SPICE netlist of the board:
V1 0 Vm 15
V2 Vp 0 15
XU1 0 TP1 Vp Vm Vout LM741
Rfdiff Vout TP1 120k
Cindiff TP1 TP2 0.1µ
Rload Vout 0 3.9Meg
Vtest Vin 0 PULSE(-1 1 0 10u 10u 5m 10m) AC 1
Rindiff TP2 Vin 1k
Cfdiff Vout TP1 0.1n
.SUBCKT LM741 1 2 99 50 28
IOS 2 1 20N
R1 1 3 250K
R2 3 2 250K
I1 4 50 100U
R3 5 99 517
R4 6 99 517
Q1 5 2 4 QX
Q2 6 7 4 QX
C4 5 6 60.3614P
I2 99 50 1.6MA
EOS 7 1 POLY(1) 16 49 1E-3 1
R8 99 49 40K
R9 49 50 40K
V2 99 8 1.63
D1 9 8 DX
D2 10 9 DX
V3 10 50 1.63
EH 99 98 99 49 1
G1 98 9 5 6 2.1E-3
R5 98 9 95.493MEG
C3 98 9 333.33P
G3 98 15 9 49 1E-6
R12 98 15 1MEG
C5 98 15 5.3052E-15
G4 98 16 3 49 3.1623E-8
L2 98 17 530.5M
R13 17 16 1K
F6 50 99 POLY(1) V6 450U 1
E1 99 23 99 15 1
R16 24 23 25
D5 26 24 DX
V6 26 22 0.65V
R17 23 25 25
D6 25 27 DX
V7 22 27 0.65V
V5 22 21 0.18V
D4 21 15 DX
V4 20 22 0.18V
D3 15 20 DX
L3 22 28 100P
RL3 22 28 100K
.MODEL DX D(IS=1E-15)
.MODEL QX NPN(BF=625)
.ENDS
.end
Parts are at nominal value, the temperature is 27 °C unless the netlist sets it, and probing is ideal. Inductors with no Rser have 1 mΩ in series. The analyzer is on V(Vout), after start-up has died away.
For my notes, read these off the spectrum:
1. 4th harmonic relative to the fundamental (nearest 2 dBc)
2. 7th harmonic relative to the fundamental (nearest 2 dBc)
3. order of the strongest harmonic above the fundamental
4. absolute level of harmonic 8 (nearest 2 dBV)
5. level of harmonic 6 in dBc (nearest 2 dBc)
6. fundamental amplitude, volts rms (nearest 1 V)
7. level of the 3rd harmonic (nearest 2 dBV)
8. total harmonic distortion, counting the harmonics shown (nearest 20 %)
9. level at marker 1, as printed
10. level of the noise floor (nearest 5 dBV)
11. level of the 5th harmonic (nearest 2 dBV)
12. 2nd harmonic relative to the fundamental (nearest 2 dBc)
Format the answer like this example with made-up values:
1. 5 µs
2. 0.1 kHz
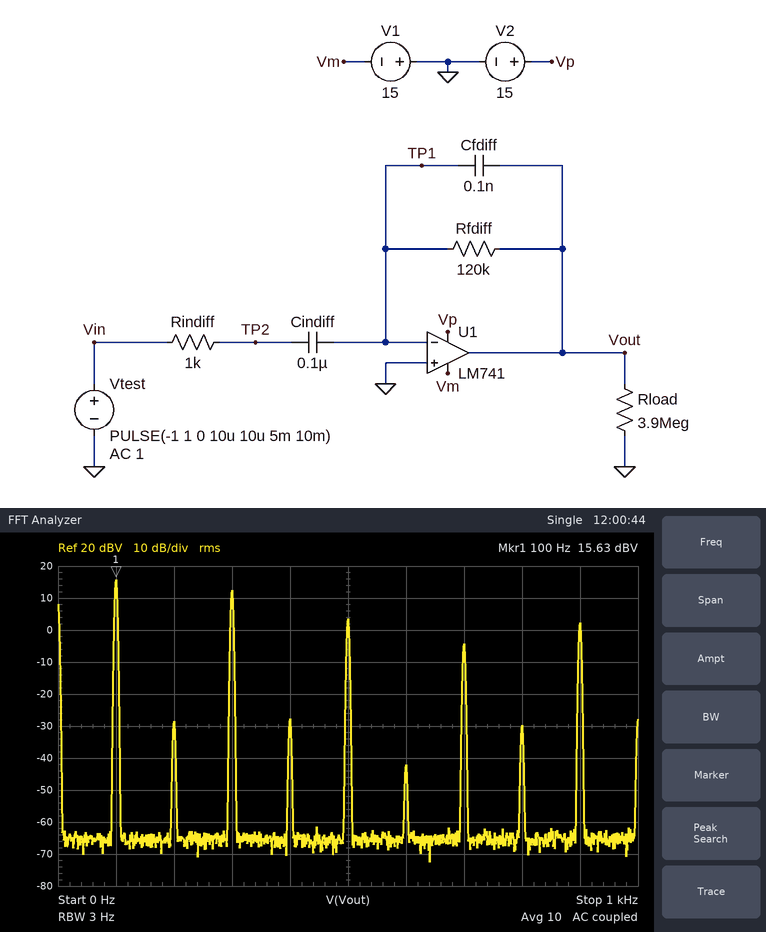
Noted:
1. -44 dBc
2. -20 dBc
3. 3
4. -30 dBV
5. -58 dBc
6. 6 V
7. 12 dBV
8. 80 %
9. 15.63 dBV
10. -65 dBV
11. 4 dBV
12. -44 dBc
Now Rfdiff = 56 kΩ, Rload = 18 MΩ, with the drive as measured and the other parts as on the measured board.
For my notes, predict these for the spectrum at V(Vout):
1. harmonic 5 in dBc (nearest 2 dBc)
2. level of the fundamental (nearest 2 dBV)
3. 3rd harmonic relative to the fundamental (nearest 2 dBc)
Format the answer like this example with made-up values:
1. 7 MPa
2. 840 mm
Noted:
1. -2 dBc
2. 10 dBV
3. 0 dBc
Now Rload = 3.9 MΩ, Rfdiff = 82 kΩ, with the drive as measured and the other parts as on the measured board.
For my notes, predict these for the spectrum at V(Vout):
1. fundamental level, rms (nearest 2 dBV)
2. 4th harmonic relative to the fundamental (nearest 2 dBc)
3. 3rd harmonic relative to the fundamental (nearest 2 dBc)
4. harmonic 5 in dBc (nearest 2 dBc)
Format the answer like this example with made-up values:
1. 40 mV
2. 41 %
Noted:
1. 12 dBV
2. -40 dBc
3. -2 dBc
4. -4 dBc
